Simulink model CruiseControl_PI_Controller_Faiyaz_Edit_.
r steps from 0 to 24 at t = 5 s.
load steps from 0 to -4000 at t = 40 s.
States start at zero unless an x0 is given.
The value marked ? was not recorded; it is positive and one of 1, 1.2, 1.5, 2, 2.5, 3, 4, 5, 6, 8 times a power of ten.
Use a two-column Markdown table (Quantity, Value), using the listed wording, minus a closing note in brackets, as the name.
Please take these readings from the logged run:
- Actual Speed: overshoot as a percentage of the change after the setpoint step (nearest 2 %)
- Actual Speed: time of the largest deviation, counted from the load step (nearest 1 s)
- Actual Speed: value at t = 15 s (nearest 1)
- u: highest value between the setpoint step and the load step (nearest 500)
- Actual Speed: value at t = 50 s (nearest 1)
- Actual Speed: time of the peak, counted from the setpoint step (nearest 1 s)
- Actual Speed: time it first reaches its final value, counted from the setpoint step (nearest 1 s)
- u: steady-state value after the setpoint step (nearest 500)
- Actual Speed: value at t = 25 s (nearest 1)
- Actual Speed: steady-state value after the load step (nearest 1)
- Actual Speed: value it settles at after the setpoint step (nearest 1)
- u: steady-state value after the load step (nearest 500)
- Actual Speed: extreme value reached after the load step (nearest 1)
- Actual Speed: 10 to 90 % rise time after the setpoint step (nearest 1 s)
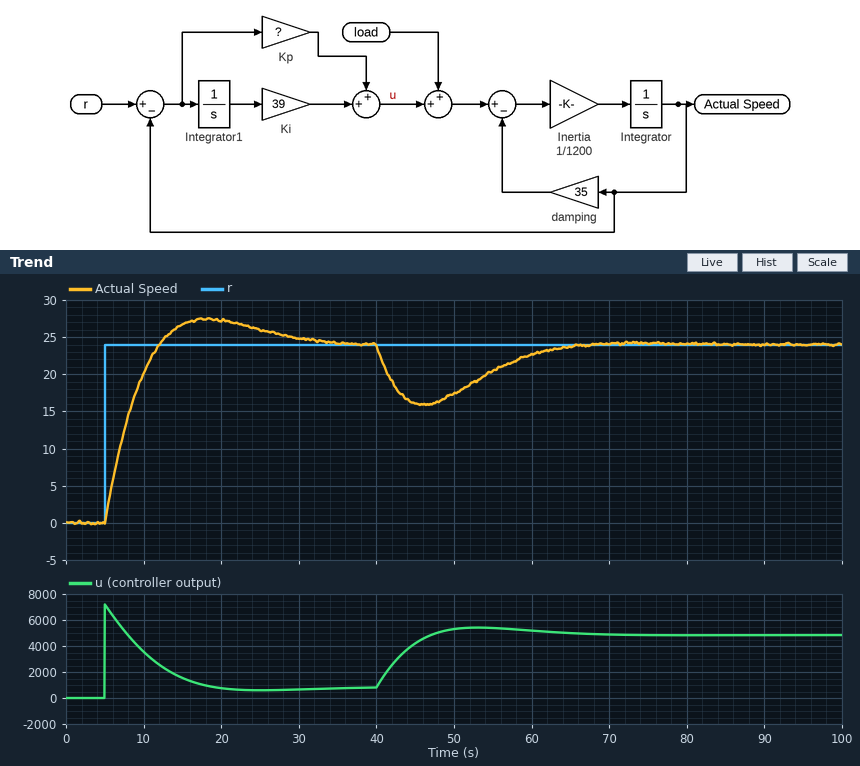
| Quantity | Value |
|---|---|
| Actual Speed: overshoot as a percentage of the change after the setpoint step | 14 % |
| Actual Speed: time of the largest deviation, counted from the load step | 6 s |
| Actual Speed: value at t = 15 s | 27 |
| u: highest value between the setpoint step and the load step | 7000 |
| Actual Speed: value at t = 50 s | 17 |
| Actual Speed: time of the peak, counted from the setpoint step | 13 s |
| Actual Speed: time it first reaches its final value, counted from the setpoint step | 7 s |
| u: steady-state value after the setpoint step | 1000 |
| Actual Speed: value at t = 25 s | 26 |
| Actual Speed: steady-state value after the load step | 24 |
| Actual Speed: value it settles at after the setpoint step | 24 |
| u: steady-state value after the load step | 5000 |
| Actual Speed: extreme value reached after the load step | 16 |
| Actual Speed: 10 to 90 % rise time after the setpoint step | 5 s |
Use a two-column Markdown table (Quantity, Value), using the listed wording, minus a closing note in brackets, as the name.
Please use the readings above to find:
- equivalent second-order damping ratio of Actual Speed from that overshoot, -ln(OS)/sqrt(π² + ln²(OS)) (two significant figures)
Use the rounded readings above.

| Quantity | Value |
|---|---|
| equivalent second-order damping ratio of Actual Speed from that overshoot, -ln(OS)/sqrt(π² + ln²(OS)) | 0.53 |
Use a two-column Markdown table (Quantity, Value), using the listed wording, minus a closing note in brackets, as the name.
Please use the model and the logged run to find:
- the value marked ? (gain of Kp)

| Quantity | Value |
|---|---|
| the value marked ? | 300 |
